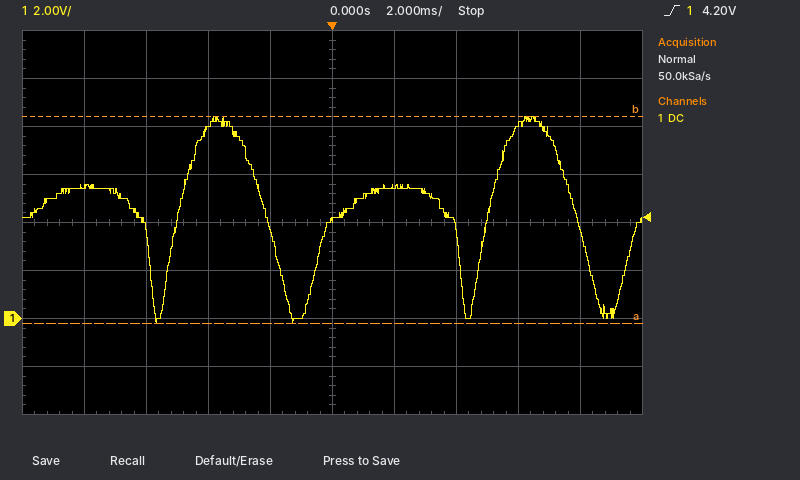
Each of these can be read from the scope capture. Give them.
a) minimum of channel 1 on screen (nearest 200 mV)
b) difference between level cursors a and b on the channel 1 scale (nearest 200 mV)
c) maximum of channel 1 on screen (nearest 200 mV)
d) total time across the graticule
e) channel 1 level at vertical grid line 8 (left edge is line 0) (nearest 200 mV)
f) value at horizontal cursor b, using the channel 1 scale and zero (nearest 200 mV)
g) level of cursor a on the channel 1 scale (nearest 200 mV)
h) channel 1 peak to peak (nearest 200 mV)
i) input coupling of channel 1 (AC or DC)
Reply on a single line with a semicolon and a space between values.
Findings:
-200 mV; 8.6 V; 8.4 V; 20 ms; 8.0 V; 8.4 V; -200 mV; 8.6 V; DC
